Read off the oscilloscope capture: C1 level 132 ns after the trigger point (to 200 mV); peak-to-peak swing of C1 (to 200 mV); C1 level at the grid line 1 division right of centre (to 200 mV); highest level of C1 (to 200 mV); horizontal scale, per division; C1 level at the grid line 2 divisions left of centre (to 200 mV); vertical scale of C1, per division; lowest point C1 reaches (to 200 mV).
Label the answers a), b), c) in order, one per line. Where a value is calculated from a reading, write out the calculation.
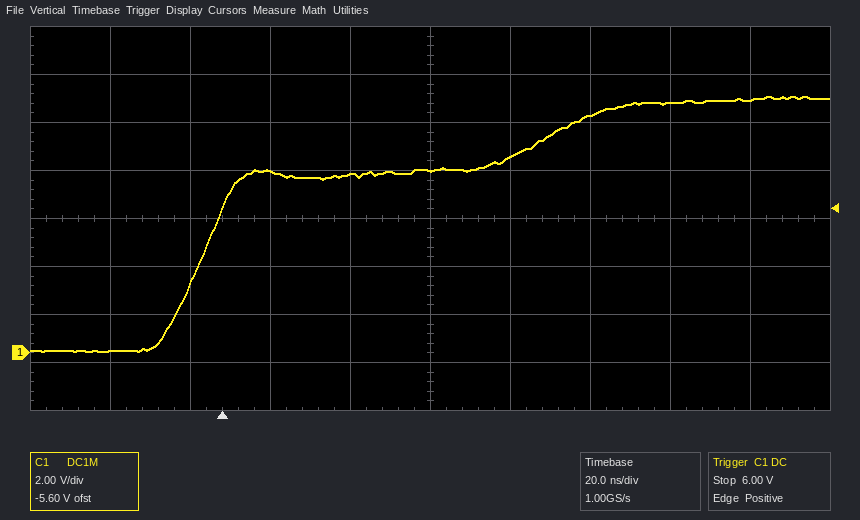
a) 10.6 V
b) 10.6 V − (0.0 V) = 10.6 V
c) 8.2 V
d) 10.6 V
e) 20 ns
f) 7.6 V
g) 2 V
h) 0.0 V
